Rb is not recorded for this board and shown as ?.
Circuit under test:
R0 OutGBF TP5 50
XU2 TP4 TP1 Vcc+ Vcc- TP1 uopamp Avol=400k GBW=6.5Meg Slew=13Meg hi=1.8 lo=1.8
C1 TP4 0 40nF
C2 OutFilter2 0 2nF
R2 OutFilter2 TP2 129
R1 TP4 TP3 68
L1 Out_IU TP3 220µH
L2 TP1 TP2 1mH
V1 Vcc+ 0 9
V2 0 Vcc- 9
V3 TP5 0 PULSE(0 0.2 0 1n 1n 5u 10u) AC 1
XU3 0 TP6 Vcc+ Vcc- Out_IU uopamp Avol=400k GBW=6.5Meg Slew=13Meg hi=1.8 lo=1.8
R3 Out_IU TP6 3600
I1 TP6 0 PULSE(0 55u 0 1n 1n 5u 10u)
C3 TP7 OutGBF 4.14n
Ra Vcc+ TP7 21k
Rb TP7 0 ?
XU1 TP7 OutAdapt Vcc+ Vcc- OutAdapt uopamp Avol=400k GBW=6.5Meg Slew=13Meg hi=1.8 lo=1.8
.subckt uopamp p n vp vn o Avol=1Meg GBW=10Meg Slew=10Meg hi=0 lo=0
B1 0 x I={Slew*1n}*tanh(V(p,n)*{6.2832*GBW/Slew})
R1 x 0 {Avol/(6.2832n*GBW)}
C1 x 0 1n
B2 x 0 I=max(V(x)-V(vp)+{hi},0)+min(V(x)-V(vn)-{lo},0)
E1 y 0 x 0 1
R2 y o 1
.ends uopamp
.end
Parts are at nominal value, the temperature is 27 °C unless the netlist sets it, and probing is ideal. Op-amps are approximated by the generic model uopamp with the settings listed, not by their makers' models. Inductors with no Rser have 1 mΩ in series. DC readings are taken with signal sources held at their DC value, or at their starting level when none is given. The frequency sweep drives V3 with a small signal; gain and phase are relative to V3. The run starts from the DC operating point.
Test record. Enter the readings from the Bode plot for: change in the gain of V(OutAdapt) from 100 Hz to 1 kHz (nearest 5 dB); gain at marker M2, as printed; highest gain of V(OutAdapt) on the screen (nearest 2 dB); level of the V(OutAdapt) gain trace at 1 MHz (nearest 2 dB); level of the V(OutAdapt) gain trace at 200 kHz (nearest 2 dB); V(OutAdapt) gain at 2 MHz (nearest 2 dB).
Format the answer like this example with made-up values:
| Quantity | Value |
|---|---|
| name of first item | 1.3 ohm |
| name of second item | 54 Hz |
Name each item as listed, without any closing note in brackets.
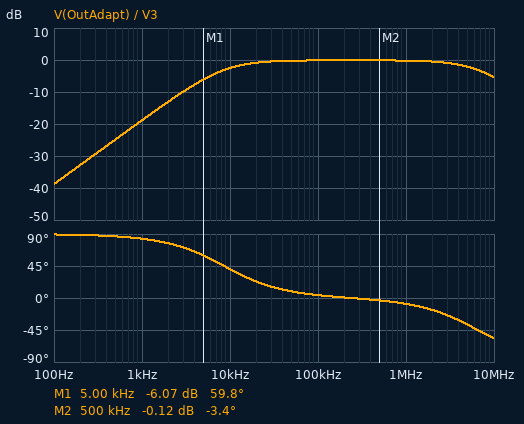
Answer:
| Quantity | Value |
|---|---|
| change in the gain of V(OutAdapt) from 100 Hz to 1 kHz | 20 dB |
| gain at marker M2, as printed | -0.12 dB |
| highest gain of V(OutAdapt) on the screen | 0 dB |
| level of the V(OutAdapt) gain trace at 1 MHz | 0 dB |
| level of the V(OutAdapt) gain trace at 200 kHz | 0 dB |
| V(OutAdapt) gain at 2 MHz | 0 dB |
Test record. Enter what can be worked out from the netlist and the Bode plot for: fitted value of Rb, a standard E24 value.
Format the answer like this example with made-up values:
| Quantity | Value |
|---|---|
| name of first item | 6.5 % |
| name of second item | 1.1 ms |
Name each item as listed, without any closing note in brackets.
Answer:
| Quantity | Value |
|---|---|
| fitted value of Rb, a standard E24 value | 5.6 kΩ |
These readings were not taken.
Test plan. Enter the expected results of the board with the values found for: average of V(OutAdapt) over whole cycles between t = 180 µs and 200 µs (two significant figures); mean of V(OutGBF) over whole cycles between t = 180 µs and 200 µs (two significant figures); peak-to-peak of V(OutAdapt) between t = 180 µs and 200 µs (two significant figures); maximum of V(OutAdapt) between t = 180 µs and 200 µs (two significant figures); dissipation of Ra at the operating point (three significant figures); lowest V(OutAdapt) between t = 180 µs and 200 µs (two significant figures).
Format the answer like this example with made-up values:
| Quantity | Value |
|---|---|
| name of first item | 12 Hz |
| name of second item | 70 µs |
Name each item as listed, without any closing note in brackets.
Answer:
| Quantity | Value |
|---|---|
| average of V(OutAdapt) over whole cycles between t = 180 µs and 200 µs | 1.9 V |
| mean of V(OutGBF) over whole cycles between t = 180 µs and 200 µs | 100 mV |
| peak-to-peak of V(OutAdapt) between t = 180 µs and 200 µs | 220 mV |
| maximum of V(OutAdapt) between t = 180 µs and 200 µs | 2.0 V |
| dissipation of Ra at the operating point | 2.40 mW |
| lowest V(OutAdapt) between t = 180 µs and 200 µs | 1.8 V |
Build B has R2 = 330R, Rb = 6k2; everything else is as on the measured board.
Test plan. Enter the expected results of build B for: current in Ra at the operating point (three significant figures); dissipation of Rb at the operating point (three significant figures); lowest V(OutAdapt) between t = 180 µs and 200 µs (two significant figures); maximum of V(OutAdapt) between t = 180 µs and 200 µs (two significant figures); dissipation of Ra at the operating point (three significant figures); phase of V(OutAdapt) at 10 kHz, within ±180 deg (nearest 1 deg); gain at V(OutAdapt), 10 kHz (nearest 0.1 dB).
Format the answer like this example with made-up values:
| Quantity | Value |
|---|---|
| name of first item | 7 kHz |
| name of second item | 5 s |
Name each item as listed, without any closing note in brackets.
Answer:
| Quantity | Value |
|---|---|
| current in Ra at the operating point | 331 µA |
| dissipation of Rb at the operating point | 679 µW |
| lowest V(OutAdapt) between t = 180 µs and 200 µs | 1.9 V |
| maximum of V(OutAdapt) between t = 180 µs and 200 µs | 2.2 V |
| dissipation of Ra at the operating point | 2.30 mW |
| phase of V(OutAdapt) at 10 kHz, within ±180 deg | 38 deg |
| gain at V(OutAdapt), 10 kHz | -2.2 dB |
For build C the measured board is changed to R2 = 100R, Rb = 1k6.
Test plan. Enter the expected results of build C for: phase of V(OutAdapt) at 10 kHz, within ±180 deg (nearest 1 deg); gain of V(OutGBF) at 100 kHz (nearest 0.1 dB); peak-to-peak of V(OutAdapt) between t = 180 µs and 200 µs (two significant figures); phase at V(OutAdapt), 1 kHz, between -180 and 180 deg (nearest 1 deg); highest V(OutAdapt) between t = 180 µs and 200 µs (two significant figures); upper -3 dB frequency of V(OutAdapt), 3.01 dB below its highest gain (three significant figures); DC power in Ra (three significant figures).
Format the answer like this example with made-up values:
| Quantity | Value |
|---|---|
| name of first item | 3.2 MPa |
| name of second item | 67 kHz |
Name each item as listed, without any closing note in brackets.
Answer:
| Quantity | Value |
|---|---|
| phase of V(OutAdapt) at 10 kHz, within ±180 deg | 68 deg |
| gain of V(OutGBF) at 100 kHz | -0.3 dB |
| peak-to-peak of V(OutAdapt) between t = 180 µs and 200 µs | 260 mV |
| phase at V(OutAdapt), 1 kHz, between -180 and 180 deg | 88 deg |
| highest V(OutAdapt) between t = 180 µs and 200 µs | 770 mV |
| upper -3 dB frequency of V(OutAdapt), 3.01 dB below its highest gain | 6.55 MHz |
| DC power in Ra | 3.33 mW |
